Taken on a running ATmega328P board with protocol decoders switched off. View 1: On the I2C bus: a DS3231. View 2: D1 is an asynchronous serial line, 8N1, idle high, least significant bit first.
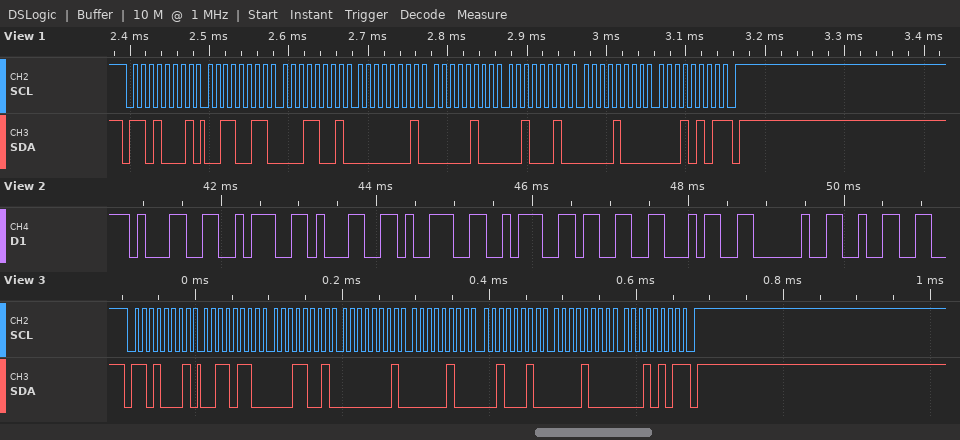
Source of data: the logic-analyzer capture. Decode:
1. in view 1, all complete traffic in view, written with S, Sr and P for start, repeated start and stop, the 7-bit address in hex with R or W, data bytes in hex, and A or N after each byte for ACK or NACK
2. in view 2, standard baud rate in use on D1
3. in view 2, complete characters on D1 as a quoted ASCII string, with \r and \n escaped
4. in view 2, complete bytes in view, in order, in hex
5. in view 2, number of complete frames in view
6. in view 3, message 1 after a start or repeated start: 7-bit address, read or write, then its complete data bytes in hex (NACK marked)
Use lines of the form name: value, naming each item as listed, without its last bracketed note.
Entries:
in view 1, all complete traffic in view, written with S, Sr and P for start, repeated start and stop, the 7-bit address in hex with R or W, data bytes in hex, and A or N after each byte for ACK or NACK: S 68R A 33 A 19 A 01 A 04 A 22 A 08 A 15 N P
in view 2, standard baud rate in use on D1: 9600 baud
in view 2, complete characters on D1 as a quoted ASCII string, with \r and \n escaped: "1:19:34 2"
in view 2, complete bytes in view, in order, in hex: 0x31 0x3A 0x31 0x39 0x3A 0x33 0x34 0x20 0x32
in view 2, number of complete frames in view: 9
in view 3, message 1 after a start or repeated start: 7-bit address, read or write, then its complete data bytes in hex: 0x68 read: 36 19 01 04 22 08 15 NACK
